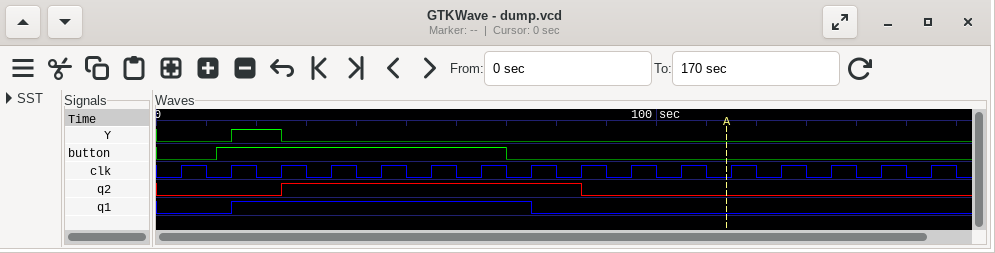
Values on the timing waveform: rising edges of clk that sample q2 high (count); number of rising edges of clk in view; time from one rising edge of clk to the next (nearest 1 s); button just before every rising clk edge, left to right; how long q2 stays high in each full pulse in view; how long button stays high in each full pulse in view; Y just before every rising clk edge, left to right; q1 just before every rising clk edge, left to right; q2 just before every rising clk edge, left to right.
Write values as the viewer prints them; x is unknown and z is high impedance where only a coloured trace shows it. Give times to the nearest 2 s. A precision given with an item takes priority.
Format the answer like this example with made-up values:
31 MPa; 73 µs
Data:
6; 16; 10 s; 0 1 1 1 1 1 1 0 0 0 0 0 0 0 0 0; 60 s; 58 s; 0 0 1 0 0 0 0 0 0 0 0 0 0 0 0 0; 0 0 1 1 1 1 1 1 0 0 0 0 0 0 0 0; 0 0 0 1 1 1 1 1 1 0 0 0 0 0 0 0
